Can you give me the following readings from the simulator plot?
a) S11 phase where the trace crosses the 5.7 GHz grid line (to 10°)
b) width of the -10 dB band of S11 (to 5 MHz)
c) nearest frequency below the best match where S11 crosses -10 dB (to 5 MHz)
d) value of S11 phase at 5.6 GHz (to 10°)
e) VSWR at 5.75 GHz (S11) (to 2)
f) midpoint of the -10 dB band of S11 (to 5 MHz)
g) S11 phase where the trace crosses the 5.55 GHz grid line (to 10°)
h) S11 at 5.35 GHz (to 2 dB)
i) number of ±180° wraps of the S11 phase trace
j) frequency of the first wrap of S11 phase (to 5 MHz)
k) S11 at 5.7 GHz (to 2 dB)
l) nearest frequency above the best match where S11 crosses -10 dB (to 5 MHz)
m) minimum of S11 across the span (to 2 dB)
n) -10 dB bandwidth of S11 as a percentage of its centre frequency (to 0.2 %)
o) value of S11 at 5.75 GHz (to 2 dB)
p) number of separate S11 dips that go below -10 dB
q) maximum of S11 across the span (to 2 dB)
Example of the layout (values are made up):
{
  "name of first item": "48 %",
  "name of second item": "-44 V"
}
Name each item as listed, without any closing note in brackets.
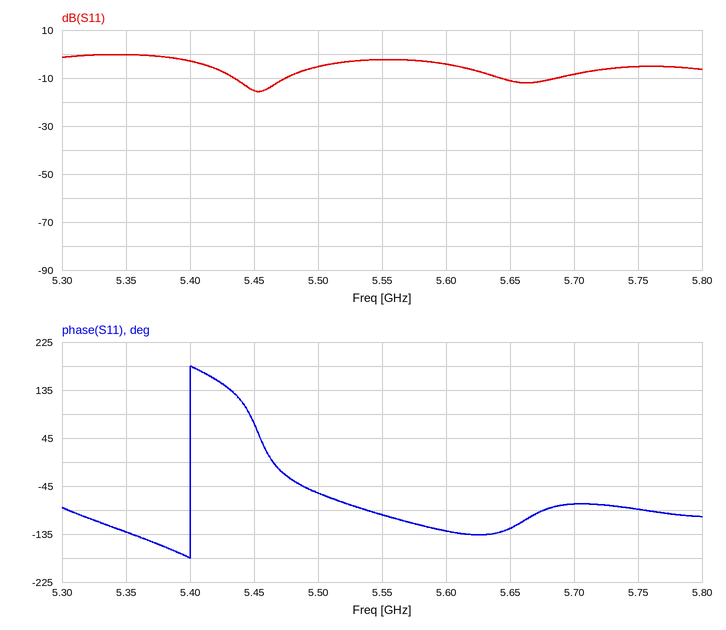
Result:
{
  "S11 phase where the trace crosses the 5.7 GHz grid line": "-80°",
  "width of the -10 dB band of S11": "40 MHz",
  "nearest frequency below the best match where S11 crosses -10 dB": "5.435 GHz",
  "value of S11 phase at 5.6 GHz": "-130°",
  "VSWR at 5.75 GHz (S11)": "4",
  "midpoint of the -10 dB band of S11": "5.455 GHz",
  "S11 phase where the trace crosses the 5.55 GHz grid line": "-100°",
  "S11 at 5.35 GHz": "0 dB",
  "number of ±180° wraps of the S11 phase trace": "1",
  "frequency of the first wrap of S11 phase": "5.400 GHz",
  "S11 at 5.7 GHz": "-8 dB",
  "nearest frequency above the best match where S11 crosses -10 dB": "5.475 GHz",
  "minimum of S11 across the span": "-16 dB",
  "-10 dB bandwidth of S11 as a percentage of its centre frequency": "0.8 %",
  "value of S11 at 5.75 GHz": "-6 dB",
  "number of separate S11 dips that go below -10 dB": "2",
  "maximum of S11 across the span": "0 dB"
}
